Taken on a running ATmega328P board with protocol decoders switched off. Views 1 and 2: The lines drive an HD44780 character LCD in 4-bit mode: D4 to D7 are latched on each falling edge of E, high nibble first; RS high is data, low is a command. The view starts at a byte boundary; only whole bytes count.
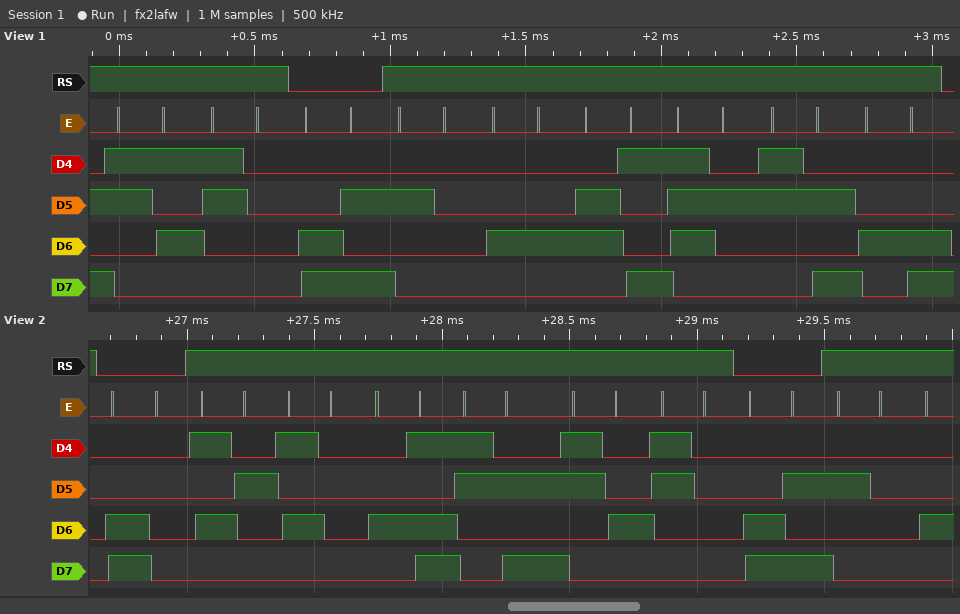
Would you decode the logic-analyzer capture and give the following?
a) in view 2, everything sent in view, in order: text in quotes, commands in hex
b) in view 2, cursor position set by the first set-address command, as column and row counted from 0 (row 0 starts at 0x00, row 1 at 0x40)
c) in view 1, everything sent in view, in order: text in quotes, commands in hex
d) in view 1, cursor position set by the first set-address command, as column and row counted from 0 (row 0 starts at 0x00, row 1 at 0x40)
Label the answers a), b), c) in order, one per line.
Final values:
a) 0xC0 "RPM:40" 0xCA " "
b) column 0, row 1
c) "50" 0xCA " Dir:L"
d) column 10, row 1
